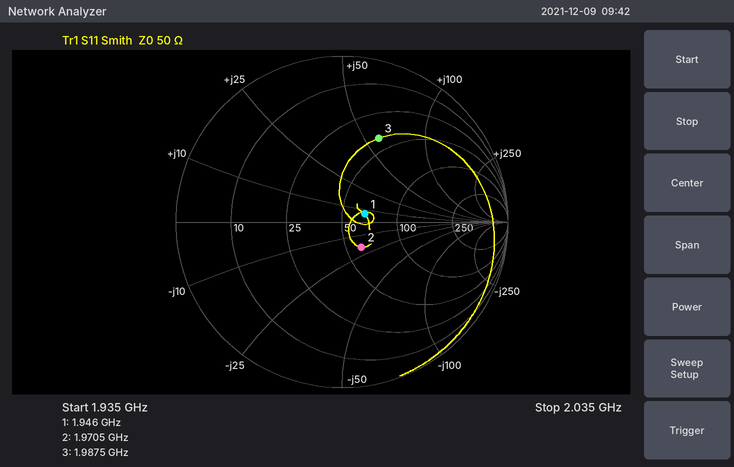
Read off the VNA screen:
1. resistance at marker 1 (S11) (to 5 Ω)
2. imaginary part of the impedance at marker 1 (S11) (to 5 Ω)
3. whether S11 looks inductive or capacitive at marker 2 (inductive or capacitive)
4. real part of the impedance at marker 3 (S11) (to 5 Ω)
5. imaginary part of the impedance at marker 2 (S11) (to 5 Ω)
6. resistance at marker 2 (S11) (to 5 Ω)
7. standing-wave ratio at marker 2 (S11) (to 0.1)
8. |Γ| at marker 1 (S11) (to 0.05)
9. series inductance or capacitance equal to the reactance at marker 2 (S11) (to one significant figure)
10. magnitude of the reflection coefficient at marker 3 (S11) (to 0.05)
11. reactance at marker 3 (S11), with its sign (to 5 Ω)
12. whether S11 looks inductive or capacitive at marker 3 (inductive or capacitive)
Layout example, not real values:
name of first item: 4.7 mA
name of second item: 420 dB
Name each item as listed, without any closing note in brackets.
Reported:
resistance at marker 1 (S11): 65 Ω
imaginary part of the impedance at marker 1 (S11): +5 Ω
whether S11 looks inductive or capacitive at marker 2: capacitive
real part of the impedance at marker 3 (S11): 40 Ω
imaginary part of the impedance at marker 2 (S11): -20 Ω
resistance at marker 2 (S11): 60 Ω
standing-wave ratio at marker 2 (S11): 1.5
|Γ| at marker 1 (S11): 0.15
series inductance or capacitance equal to the reactance at marker 2 (S11): 4 pF
magnitude of the reflection coefficient at marker 3 (S11): 0.55
reactance at marker 3 (S11), with its sign: +60 Ω
whether S11 looks inductive or capacitive at marker 3: inductive
